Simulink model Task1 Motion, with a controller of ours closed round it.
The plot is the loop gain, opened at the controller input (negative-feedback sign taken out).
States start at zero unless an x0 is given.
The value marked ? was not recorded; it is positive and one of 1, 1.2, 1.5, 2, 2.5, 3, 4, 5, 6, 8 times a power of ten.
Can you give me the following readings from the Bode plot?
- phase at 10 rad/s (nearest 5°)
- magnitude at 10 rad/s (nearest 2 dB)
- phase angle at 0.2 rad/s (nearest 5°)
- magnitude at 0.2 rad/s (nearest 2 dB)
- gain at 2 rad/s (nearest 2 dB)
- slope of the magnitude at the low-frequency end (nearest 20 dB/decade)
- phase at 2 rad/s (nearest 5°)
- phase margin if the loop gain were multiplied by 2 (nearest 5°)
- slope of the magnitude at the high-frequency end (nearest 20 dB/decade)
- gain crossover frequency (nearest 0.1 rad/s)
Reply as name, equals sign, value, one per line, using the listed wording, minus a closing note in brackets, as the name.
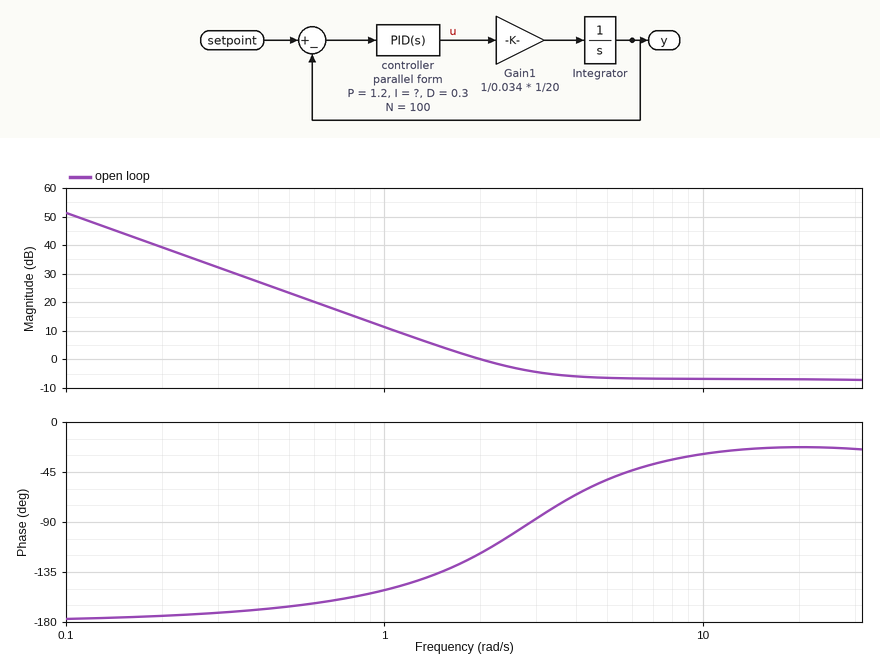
phase at 10 rad/s = -30°
magnitude at 10 rad/s = -6 dB
phase angle at 0.2 rad/s = -175°
magnitude at 0.2 rad/s = 40 dB
gain at 2 rad/s = 0 dB
slope of the magnitude at the low-frequency end = -40 dB/decade
phase at 2 rad/s = -120°
phase margin if the loop gain were multiplied by 2 = 115°
slope of the magnitude at the high-frequency end = 0 dB/decade
gain crossover frequency = 2.0 rad/s
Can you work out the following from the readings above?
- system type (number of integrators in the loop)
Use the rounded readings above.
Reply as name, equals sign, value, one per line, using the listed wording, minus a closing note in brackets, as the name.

system type = 2
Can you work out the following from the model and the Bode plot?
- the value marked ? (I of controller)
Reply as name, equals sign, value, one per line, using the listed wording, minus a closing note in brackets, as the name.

the value marked ? = 2.5
